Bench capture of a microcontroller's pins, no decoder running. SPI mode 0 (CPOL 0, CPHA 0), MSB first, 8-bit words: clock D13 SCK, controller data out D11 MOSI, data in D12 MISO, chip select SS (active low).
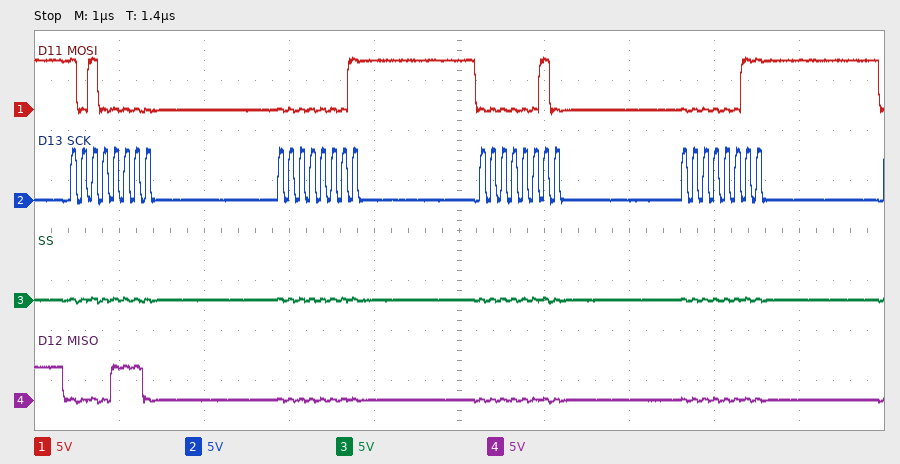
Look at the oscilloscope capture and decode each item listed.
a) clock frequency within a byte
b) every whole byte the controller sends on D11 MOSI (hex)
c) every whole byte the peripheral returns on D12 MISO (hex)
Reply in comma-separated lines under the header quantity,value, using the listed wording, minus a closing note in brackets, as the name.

quantity,value
clock frequency within a byte,8 MHz
every whole byte the controller sends on D11 MOSI,A0 01 02 03
every whole byte the peripheral returns on D12 MISO,0E 00 00 00
